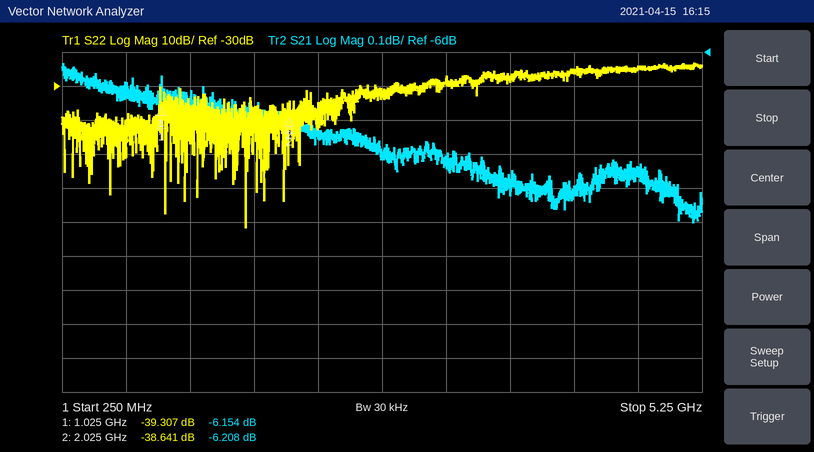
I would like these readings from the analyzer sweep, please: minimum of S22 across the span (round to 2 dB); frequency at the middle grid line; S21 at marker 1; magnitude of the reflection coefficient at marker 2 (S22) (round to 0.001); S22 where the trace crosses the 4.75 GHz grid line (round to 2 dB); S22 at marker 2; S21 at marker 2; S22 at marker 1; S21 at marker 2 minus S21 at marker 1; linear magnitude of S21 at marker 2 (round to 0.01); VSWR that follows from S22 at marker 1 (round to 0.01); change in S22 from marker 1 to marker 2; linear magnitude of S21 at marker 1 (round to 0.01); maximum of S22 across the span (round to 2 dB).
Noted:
-72 dB
2.75 GHz
-6.154 dB
0.012
-24 dB
-38.641 dB
-6.208 dB
-39.307 dB
-0.054 dB
0.49
1.02
0.666 dB
0.49
-24 dB
